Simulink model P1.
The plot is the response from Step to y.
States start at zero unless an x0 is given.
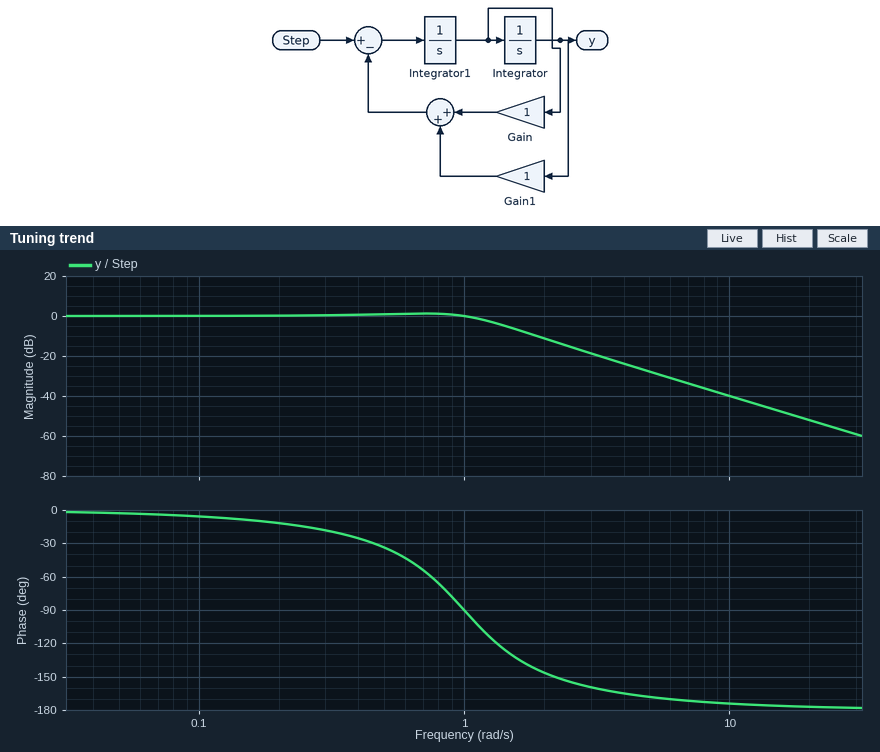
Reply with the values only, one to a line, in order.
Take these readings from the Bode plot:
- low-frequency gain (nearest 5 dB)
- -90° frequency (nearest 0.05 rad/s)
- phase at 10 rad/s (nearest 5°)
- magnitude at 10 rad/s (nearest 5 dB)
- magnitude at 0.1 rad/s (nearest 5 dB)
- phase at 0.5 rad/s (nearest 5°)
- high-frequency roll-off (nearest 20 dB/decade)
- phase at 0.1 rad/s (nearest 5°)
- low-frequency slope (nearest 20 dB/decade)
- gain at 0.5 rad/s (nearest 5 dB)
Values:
0 dB
1.00 rad/s
-175°
-40 dB
0 dB
-35°
-40 dB/decade
-5°
0 dB/decade
0 dB
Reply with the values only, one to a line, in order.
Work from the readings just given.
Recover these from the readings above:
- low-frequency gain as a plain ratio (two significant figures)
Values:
1.0
